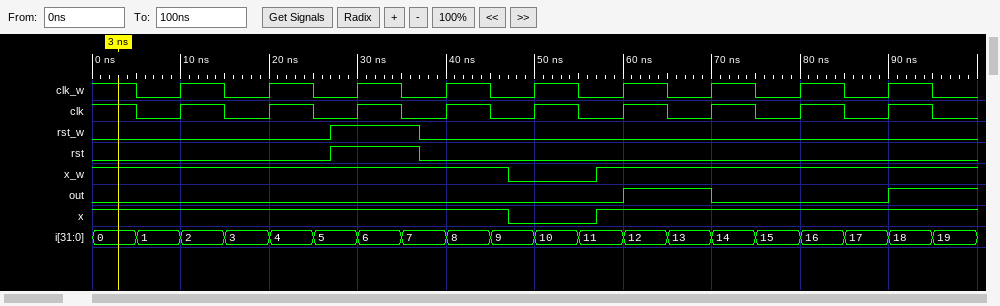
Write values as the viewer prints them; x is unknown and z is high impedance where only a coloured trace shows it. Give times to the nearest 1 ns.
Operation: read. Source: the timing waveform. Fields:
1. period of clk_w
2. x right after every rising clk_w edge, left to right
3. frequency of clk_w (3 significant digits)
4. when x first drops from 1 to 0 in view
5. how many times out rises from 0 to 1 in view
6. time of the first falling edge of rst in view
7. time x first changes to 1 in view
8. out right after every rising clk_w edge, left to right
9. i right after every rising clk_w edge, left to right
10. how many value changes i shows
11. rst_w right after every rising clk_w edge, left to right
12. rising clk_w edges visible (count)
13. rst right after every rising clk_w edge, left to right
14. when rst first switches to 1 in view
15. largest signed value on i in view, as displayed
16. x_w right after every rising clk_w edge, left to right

10 ns
1 1 1 1 0 1 1 1 1
100 MHz
47 ns
2
37 ns
57 ns
0 0 0 0 0 1 0 0 1
2, 4, 6, 8, 10, 12, 14, 16, 18
19
0 0 1 0 0 0 0 0 0
9
0 0 1 0 0 0 0 0 0
27 ns
19
1 1 1 1 0 1 1 1 1
